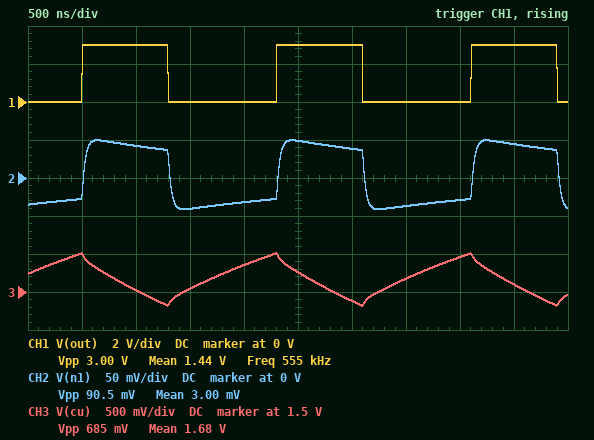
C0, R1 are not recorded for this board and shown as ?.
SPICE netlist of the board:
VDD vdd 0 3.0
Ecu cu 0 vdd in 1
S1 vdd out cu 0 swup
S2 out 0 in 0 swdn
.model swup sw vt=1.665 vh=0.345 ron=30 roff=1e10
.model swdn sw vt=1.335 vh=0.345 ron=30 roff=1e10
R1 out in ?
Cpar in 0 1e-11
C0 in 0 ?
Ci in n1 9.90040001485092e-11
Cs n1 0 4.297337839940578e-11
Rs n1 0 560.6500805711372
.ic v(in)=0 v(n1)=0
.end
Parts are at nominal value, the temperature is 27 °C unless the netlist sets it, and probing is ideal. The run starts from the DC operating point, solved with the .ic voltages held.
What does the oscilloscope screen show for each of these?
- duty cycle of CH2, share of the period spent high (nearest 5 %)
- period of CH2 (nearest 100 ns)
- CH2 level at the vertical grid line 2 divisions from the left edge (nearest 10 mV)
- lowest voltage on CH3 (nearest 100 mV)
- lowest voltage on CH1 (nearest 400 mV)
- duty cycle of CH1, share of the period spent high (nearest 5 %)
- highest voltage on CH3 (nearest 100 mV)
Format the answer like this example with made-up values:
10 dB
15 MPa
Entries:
45 %
1.8 µs
40 mV
1.3 V
0 V
45 %
2.0 V
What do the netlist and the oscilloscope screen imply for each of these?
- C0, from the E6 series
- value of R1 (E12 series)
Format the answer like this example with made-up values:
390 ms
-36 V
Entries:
3.3 pF
18 kΩ
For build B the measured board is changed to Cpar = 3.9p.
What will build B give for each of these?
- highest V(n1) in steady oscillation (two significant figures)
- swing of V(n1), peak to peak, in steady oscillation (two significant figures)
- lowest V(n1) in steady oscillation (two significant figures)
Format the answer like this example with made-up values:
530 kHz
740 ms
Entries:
52 mV
96 mV
-43 mV
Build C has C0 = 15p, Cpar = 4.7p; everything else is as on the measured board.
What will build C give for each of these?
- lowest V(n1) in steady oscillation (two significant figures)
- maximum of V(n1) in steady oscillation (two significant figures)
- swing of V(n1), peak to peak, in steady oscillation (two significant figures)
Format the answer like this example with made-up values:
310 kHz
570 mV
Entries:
-39 mV
47 mV
86 mV
